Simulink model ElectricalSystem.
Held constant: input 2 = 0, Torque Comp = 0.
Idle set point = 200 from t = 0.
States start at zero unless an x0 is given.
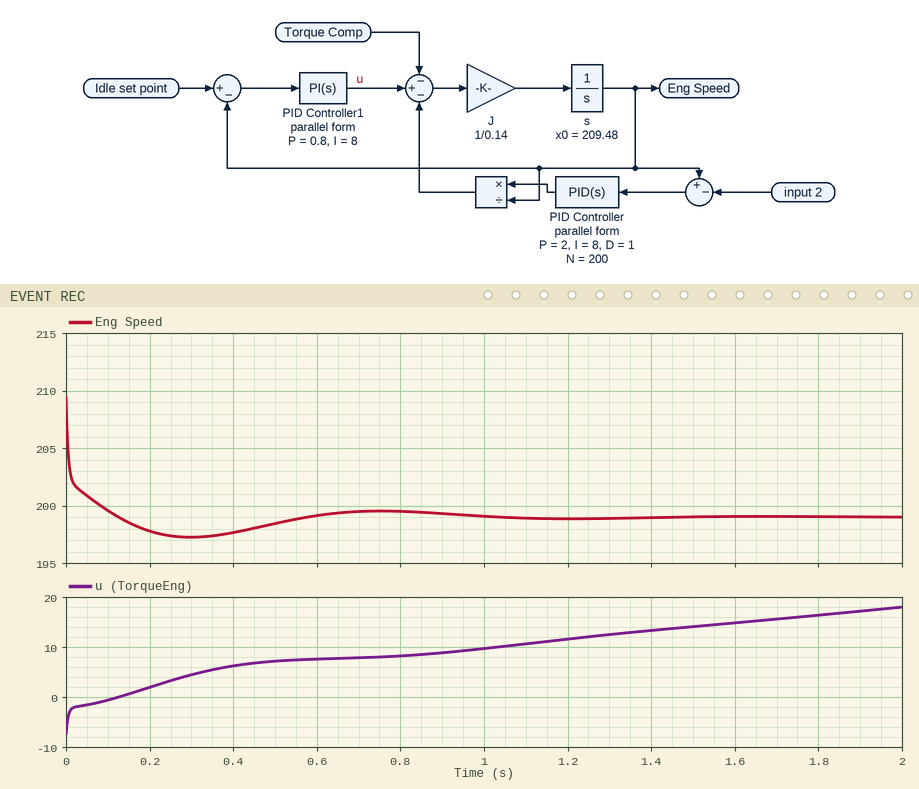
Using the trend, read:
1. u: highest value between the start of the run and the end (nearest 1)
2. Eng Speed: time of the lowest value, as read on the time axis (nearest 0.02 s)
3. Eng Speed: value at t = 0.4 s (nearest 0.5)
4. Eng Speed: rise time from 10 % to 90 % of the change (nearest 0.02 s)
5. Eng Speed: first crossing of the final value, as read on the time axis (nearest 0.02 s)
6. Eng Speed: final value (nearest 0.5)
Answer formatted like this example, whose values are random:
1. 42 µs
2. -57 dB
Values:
1. 18
2. 0.30 s
3. 197.5
4. 0.08 s
5. 0.12 s
6. 199.0
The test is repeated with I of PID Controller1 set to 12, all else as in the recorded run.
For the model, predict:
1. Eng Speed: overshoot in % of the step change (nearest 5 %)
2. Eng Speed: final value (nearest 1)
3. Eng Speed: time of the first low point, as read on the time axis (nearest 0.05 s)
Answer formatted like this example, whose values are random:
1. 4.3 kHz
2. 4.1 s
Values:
1. 20 %
2. 199
3. 0.25 s
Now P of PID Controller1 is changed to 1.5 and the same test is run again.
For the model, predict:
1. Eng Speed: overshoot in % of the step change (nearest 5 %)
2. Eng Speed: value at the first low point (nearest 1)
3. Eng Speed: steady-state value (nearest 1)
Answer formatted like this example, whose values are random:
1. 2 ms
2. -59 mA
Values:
1. 10 %
2. 198
3. 199
